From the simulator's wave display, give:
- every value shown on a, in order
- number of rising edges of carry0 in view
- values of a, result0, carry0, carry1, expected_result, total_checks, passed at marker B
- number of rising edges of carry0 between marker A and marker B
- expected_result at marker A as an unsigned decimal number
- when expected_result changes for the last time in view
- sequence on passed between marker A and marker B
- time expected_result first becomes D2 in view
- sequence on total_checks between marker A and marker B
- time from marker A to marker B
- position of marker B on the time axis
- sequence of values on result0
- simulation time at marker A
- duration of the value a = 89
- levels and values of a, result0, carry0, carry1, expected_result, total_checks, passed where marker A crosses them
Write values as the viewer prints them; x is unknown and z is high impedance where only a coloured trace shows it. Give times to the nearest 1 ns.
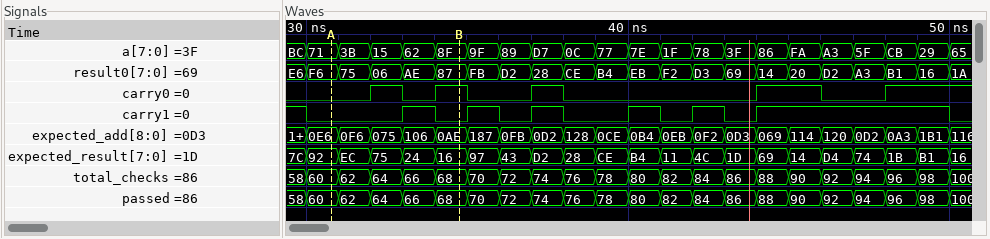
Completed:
BC, 71, 3B, 15, 62, 8F, 9F, 89, D7, 0C, 77, 7E, 1F, 78, 3F, 86, FA, A3, 5F, CB, 29, 65
5
a=8F, result0=87, carry0=1, carry1=0, expected_result=16, total_checks=68, passed=68
2
146
50 ns
60, 62, 64, 66, 68
37 ns
60, 62, 64, 66, 68
4 ns
35 ns
E6, F6, 75, 06, AE, 87, FB, D2, 28, CE, B4, EB, F2, D3, 69, 14, 20, D2, A3, B1, 16, 1A
31 ns
1 ns
a=71, result0=F6, carry0=0, carry1=0, expected_result=92, total_checks=60, passed=60
